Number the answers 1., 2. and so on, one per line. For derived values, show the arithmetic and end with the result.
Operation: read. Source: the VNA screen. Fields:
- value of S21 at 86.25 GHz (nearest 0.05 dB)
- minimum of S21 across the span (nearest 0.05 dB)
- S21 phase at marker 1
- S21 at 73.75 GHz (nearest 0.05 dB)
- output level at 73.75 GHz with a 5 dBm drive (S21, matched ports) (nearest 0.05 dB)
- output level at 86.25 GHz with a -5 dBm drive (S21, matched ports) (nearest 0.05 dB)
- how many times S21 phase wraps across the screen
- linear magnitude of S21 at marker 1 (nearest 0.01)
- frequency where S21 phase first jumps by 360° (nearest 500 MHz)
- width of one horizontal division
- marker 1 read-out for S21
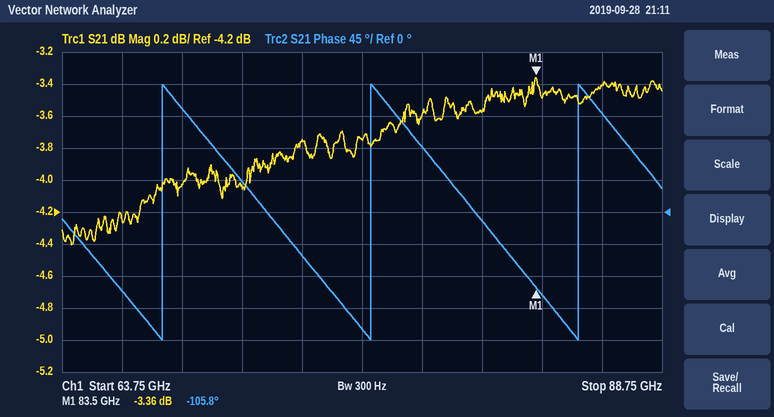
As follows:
1. -3.40 dB
2. -4.40 dB
3. -105.8°
4. -3.75 dB
5. 5 dBm + (-3.75 dB) = 1.25 dBm
6. -5 dBm + (-3.40 dB) = -8.40 dBm
7. 3
8. 10^(-3.36/20) ≈ 0.68
9. 68.0 GHz
10. 2.5 GHz
11. -3.36 dB
